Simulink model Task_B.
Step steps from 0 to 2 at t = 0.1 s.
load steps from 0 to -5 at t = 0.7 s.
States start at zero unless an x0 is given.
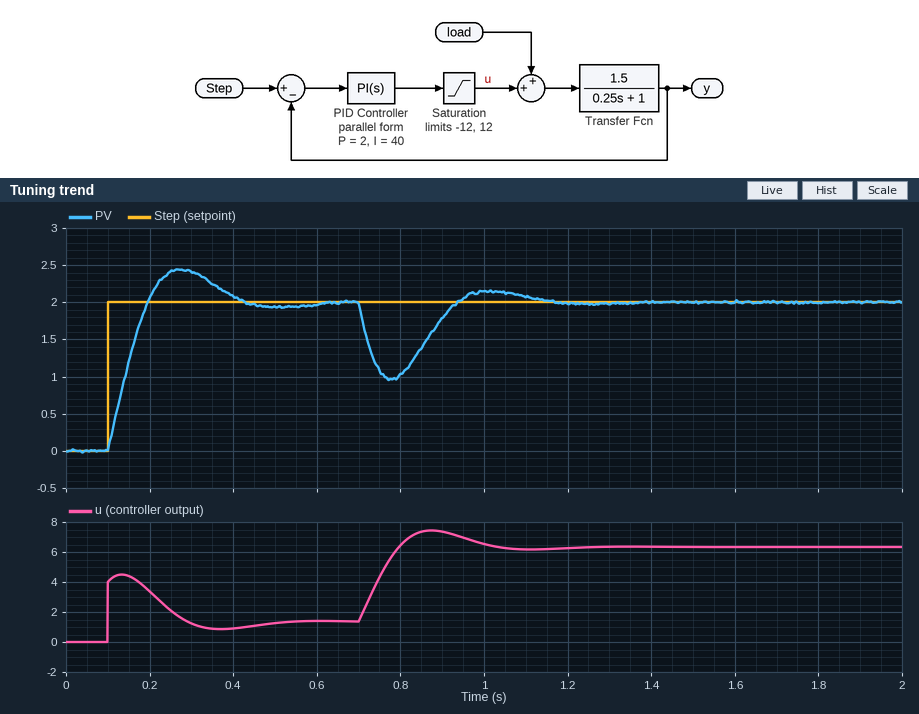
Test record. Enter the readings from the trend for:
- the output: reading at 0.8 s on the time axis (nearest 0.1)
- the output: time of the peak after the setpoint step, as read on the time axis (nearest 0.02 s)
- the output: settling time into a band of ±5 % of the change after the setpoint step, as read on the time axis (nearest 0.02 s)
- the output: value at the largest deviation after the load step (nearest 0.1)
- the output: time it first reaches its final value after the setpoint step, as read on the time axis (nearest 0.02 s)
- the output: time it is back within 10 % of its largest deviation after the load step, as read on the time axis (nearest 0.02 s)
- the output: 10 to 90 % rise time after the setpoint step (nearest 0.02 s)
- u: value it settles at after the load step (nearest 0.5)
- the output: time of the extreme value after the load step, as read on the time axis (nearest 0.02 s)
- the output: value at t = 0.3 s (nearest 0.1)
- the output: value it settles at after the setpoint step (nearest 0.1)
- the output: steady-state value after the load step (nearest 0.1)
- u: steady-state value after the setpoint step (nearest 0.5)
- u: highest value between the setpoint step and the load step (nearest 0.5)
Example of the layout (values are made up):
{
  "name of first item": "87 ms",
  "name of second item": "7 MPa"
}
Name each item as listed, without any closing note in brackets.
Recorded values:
{
  "the output: reading at 0.8 s on the time axis": "1.0",
  "the output: time of the peak after the setpoint step, as read on the time axis": "0.28 s",
  "the output: settling time into a band of ±5 % of the change after the setpoint step, as read on the time axis": "0.40 s",
  "the output: value at the largest deviation after the load step": "1.0",
  "the output: time it first reaches its final value after the setpoint step, as read on the time axis": "0.20 s",
  "the output: time it is back within 10 % of its largest deviation after the load step, as read on the time axis": "1.08 s",
  "the output: 10 to 90 % rise time after the setpoint step": "0.08 s",
  "u: value it settles at after the load step": "6.5",
  "the output: time of the extreme value after the load step, as read on the time axis": "0.78 s",
  "the output: value at t = 0.3 s": "2.4",
  "the output: value it settles at after the setpoint step": "2.0",
  "the output: steady-state value after the load step": "2.0",
  "u: steady-state value after the setpoint step": "1.5",
  "u: highest value between the setpoint step and the load step": "4.5"
}
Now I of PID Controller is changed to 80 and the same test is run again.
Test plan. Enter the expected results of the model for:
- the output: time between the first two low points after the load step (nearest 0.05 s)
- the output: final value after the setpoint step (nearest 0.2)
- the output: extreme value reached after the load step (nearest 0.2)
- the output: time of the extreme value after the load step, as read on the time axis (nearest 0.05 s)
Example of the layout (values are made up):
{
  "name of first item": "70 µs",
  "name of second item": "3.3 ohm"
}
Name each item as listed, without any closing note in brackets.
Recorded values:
{
  "the output: time between the first two low points after the load step": "0.30 s",
  "the output: final value after the setpoint step": "2.0",
  "the output: extreme value reached after the load step": "1.2",
  "the output: time of the extreme value after the load step, as read on the time axis": "0.75 s"
}
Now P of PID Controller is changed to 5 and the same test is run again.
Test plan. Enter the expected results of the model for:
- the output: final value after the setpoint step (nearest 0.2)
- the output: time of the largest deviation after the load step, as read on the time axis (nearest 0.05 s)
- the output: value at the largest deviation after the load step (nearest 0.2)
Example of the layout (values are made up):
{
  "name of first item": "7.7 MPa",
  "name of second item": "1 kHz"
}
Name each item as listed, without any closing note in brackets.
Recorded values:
{
  "the output: final value after the setpoint step": "2.0",
  "the output: time of the largest deviation after the load step, as read on the time axis": "0.75 s",
  "the output: value at the largest deviation after the load step": "1.4"
}
